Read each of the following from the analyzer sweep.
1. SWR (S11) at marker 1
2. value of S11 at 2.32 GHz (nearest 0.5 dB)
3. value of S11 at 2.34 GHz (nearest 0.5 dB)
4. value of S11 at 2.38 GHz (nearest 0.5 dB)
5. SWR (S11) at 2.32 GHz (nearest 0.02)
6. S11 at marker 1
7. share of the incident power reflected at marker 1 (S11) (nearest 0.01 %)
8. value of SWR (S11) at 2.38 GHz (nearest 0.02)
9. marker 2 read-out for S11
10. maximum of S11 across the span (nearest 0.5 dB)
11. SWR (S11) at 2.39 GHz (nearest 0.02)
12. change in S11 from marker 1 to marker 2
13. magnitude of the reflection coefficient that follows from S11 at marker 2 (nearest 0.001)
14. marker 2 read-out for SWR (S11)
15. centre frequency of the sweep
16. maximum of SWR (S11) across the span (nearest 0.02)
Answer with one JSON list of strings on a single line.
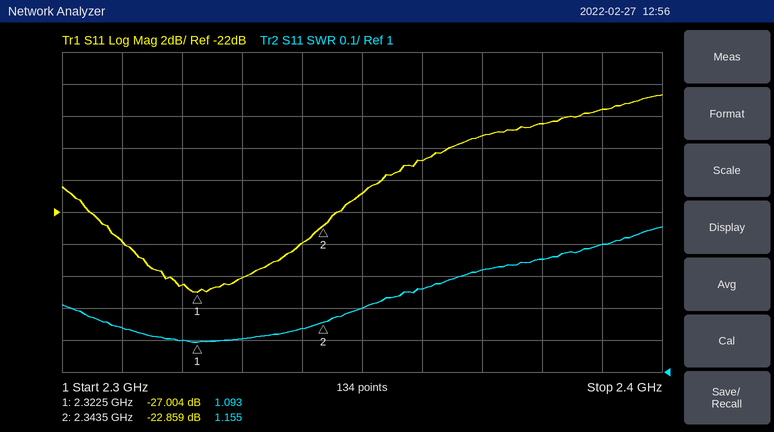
["1.093", "-26.5 dB", "-24.0 dB", "-16.5 dB", "1.10", "-27.004 dB", "0.20 %", "1.36", "-22.859 dB", "-14.5 dB", "1.40", "4.145 dB", "0.072", "1.155", "2.35 GHz", "1.46"]
